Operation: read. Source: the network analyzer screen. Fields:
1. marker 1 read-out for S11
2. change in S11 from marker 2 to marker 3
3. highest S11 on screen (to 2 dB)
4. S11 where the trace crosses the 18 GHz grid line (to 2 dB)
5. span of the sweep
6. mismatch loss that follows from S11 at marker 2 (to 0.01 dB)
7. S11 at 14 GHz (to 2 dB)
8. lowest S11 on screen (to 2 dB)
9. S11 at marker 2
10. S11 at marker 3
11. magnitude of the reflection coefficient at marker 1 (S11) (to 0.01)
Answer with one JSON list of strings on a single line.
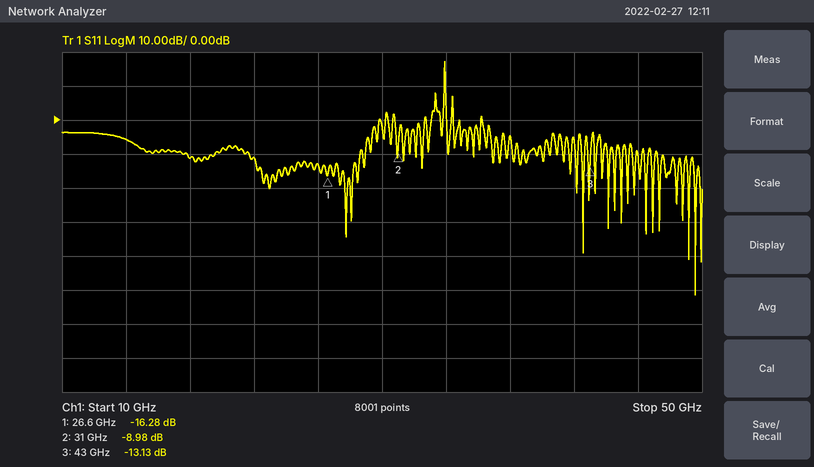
["-16.28 dB", "-4.15 dB", "18 dB", "-12 dB", "40 GHz", "0.59 dB", "-6 dB", "-52 dB", "-8.98 dB", "-13.13 dB", "0.15"]
